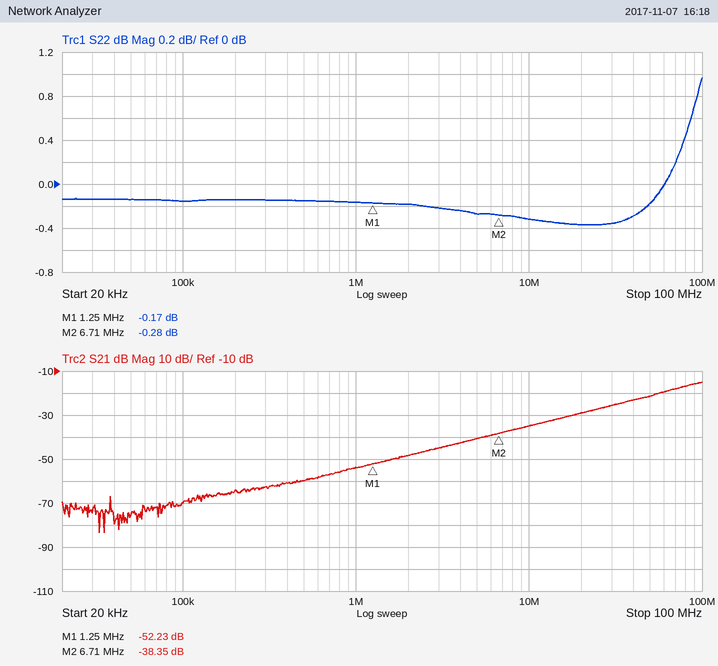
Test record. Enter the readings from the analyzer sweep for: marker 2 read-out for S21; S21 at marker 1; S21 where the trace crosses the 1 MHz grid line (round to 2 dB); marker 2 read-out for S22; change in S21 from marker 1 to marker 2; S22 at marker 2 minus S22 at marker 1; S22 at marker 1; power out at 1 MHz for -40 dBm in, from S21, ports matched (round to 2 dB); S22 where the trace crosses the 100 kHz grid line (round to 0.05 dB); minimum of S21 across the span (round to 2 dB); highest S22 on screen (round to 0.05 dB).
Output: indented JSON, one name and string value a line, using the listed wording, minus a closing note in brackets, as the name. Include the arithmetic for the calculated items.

{
  "marker 2 read-out for S21": "-38.35 dB",
  "S21 at marker 1": "-52.23 dB",
  "S21 where the trace crosses the 1 MHz grid line": "-54 dB",
  "marker 2 read-out for S22": "-0.28 dB",
  "change in S21 from marker 1 to marker 2": "-38.35 − (-52.23) = 13.88 dB",
  "S22 at marker 2 minus S22 at marker 1": "-0.28 − (-0.17) = -0.11 dB",
  "S22 at marker 1": "-0.17 dB",
  "power out at 1 MHz for -40 dBm in, from S21, ports matched": "-40 dBm + (-54 dB) = -94 dBm",
  "S22 where the trace crosses the 100 kHz grid line": "-0.15 dB",
  "minimum of S21 across the span": "-84 dB",
  "highest S22 on screen": "0.95 dB"
}
